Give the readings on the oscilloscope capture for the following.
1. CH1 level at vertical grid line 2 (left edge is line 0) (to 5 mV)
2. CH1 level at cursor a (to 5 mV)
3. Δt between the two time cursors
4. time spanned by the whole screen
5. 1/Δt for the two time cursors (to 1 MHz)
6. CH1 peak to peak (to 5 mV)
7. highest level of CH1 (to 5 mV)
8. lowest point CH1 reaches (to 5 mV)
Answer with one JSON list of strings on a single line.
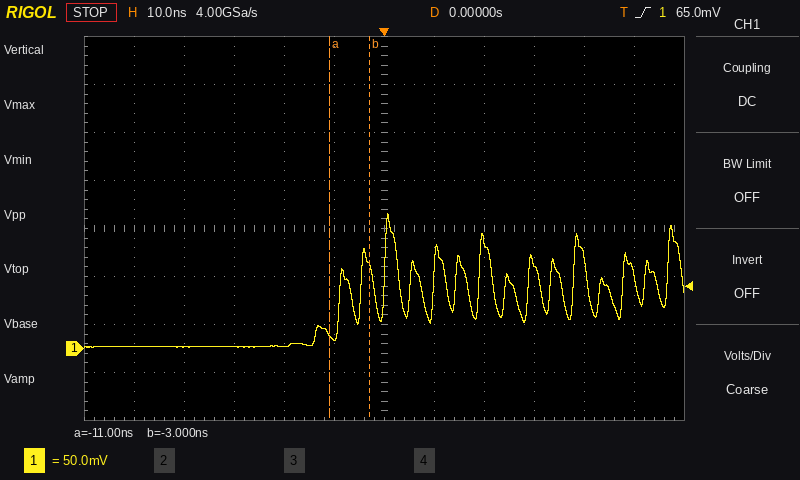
["0 mV", "15 mV", "8 ns", "120 ns", "125 MHz", "140 mV", "140 mV", "0 mV"]
